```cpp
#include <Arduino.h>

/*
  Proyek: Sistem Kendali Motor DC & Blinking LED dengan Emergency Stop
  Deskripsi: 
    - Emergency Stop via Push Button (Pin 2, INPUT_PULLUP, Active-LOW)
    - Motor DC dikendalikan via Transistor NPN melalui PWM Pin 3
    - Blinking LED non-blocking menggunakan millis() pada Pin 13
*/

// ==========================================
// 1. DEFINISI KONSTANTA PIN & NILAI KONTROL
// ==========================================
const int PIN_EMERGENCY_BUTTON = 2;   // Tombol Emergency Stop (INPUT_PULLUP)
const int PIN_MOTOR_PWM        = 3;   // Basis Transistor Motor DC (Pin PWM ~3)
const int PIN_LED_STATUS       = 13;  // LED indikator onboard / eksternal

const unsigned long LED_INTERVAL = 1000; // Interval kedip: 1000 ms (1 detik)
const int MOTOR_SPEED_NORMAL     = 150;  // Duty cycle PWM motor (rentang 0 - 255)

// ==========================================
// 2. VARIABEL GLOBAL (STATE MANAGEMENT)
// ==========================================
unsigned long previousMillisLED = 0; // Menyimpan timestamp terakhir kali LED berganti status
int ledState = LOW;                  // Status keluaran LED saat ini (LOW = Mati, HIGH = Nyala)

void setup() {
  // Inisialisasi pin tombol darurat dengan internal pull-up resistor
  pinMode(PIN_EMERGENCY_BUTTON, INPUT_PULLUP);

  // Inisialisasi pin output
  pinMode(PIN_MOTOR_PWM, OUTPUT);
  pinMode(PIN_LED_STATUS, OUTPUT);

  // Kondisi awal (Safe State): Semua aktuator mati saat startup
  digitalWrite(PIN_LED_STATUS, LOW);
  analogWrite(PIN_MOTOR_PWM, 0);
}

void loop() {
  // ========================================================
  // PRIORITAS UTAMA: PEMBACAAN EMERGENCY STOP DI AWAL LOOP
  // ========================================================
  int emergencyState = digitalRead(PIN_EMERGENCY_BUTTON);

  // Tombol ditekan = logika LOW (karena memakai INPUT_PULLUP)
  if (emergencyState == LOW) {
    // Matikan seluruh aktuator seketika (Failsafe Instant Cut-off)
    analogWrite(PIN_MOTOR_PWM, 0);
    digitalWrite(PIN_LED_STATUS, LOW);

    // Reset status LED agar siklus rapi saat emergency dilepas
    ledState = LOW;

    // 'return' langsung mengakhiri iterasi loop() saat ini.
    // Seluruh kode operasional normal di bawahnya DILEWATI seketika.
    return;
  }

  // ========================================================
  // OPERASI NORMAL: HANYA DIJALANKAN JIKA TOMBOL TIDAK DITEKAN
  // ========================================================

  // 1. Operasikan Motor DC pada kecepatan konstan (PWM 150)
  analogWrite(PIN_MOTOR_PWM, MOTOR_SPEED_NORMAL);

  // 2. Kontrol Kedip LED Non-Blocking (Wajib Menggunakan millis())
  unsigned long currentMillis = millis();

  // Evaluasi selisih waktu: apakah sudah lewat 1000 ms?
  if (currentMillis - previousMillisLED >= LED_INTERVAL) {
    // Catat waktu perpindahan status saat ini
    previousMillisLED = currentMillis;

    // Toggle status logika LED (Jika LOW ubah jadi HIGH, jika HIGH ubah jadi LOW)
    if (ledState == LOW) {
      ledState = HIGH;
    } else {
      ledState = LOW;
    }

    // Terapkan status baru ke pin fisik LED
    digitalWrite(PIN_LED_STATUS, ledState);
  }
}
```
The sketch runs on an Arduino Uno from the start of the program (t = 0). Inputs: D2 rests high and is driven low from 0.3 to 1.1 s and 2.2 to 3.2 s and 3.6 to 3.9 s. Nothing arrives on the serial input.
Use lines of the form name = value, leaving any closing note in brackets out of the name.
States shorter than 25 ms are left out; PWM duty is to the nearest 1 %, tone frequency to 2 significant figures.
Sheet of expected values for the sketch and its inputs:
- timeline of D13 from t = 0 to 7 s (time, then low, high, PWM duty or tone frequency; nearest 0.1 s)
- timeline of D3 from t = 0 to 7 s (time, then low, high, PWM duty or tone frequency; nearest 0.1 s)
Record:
timeline of D13 from t = 0 to 7 s = 0 s low; 1.1 s high; 2.1 s low; 3.2 s high; 3.6 s low; 4.2 s high; 5.2 s low; 6.2 s high
timeline of D3 from t = 0 to 7 s = 0 s PWM 59 %; 0.3 s low; 1.1 s PWM 59 %; 2.2 s low; 3.2 s PWM 59 %; 3.6 s low; 3.9 s PWM 59 %
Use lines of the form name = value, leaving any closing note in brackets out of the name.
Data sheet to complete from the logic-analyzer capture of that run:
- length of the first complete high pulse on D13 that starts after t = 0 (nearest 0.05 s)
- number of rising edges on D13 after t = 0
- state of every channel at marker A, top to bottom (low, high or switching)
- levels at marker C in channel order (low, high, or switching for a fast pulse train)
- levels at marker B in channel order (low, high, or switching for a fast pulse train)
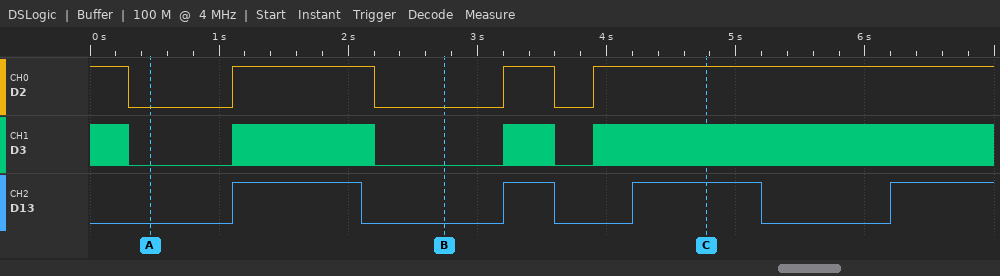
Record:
length of the first complete high pulse on D13 that starts after t = 0 = 1.00 s
number of rising edges on D13 after t = 0 = 4
state of every channel at marker A, top to bottom = D2 low, D3 low, D13 low
levels at marker C in channel order = D2 high, D3 switching, D13 high
levels at marker B in channel order = D2 low, D3 low, D13 low
